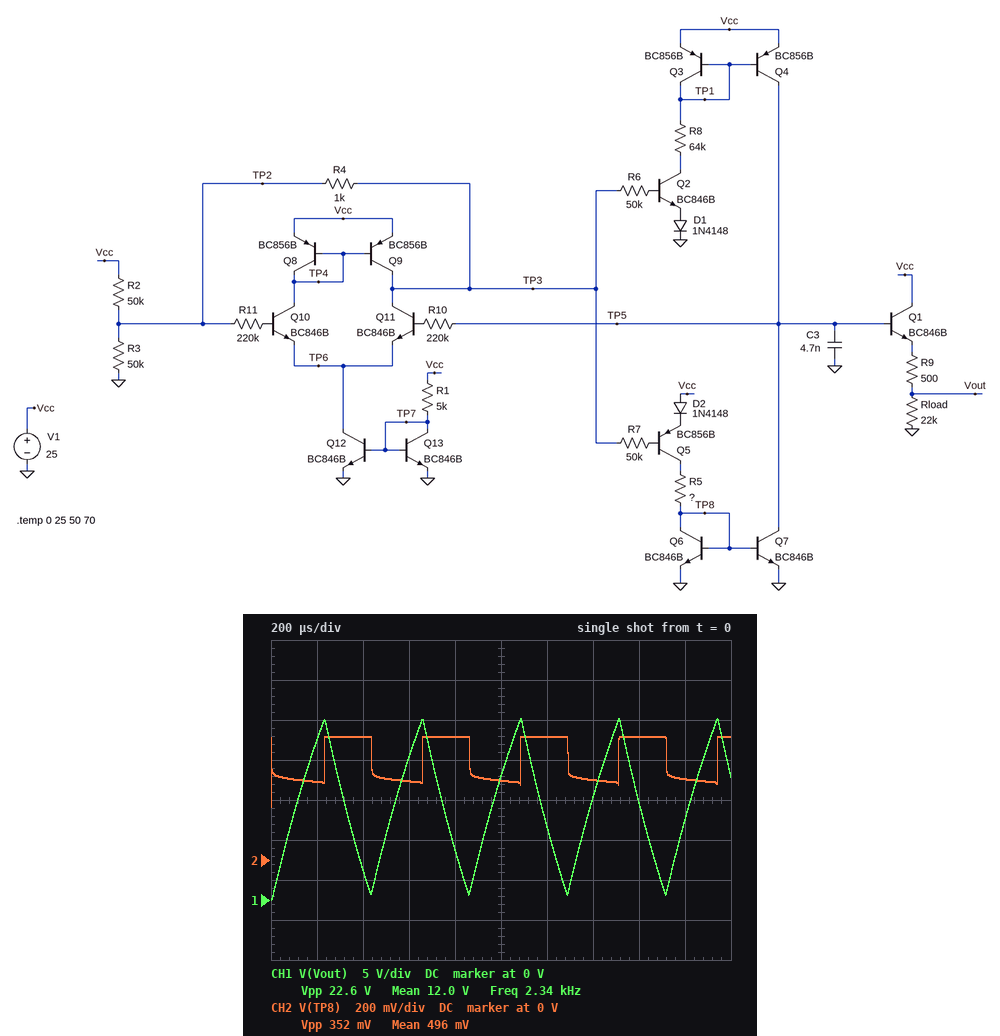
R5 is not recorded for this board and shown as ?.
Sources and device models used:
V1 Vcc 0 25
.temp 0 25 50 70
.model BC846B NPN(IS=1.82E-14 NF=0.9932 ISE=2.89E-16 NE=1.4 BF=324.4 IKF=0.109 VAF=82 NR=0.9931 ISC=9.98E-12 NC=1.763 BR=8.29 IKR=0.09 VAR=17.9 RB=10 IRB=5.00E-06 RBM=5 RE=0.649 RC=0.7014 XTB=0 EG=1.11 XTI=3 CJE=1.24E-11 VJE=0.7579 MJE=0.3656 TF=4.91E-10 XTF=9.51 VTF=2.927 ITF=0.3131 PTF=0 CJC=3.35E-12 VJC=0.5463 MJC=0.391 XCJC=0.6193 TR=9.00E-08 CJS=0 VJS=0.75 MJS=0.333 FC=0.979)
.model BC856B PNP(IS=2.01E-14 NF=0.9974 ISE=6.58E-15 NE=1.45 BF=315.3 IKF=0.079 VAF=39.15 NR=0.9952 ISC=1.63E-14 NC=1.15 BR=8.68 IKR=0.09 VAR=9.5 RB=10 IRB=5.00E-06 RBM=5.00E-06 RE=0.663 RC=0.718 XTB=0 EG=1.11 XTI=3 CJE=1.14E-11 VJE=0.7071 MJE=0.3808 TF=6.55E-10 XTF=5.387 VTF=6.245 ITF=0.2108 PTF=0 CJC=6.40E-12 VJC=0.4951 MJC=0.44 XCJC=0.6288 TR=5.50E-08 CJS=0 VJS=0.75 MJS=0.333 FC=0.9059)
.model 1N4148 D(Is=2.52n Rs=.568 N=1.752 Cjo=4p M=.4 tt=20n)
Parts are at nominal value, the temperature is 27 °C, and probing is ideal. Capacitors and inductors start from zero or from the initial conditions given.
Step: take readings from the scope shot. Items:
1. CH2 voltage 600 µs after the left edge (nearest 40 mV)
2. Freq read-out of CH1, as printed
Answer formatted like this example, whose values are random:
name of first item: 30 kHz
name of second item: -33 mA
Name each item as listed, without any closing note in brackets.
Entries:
CH2 voltage 600 µs after the left edge: 400 mV
Freq read-out of CH1, as printed: 2.34 kHz
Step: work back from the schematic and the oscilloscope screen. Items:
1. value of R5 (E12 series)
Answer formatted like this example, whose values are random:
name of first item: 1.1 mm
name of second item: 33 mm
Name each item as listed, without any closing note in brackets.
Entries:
value of R5: 56 kΩ
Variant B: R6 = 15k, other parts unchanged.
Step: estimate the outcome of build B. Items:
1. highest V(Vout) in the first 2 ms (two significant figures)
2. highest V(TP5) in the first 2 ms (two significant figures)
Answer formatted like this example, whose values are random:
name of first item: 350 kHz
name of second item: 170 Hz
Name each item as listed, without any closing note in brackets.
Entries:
highest V(Vout) in the first 2 ms: 22 V
highest V(TP5) in the first 2 ms: 23 V
